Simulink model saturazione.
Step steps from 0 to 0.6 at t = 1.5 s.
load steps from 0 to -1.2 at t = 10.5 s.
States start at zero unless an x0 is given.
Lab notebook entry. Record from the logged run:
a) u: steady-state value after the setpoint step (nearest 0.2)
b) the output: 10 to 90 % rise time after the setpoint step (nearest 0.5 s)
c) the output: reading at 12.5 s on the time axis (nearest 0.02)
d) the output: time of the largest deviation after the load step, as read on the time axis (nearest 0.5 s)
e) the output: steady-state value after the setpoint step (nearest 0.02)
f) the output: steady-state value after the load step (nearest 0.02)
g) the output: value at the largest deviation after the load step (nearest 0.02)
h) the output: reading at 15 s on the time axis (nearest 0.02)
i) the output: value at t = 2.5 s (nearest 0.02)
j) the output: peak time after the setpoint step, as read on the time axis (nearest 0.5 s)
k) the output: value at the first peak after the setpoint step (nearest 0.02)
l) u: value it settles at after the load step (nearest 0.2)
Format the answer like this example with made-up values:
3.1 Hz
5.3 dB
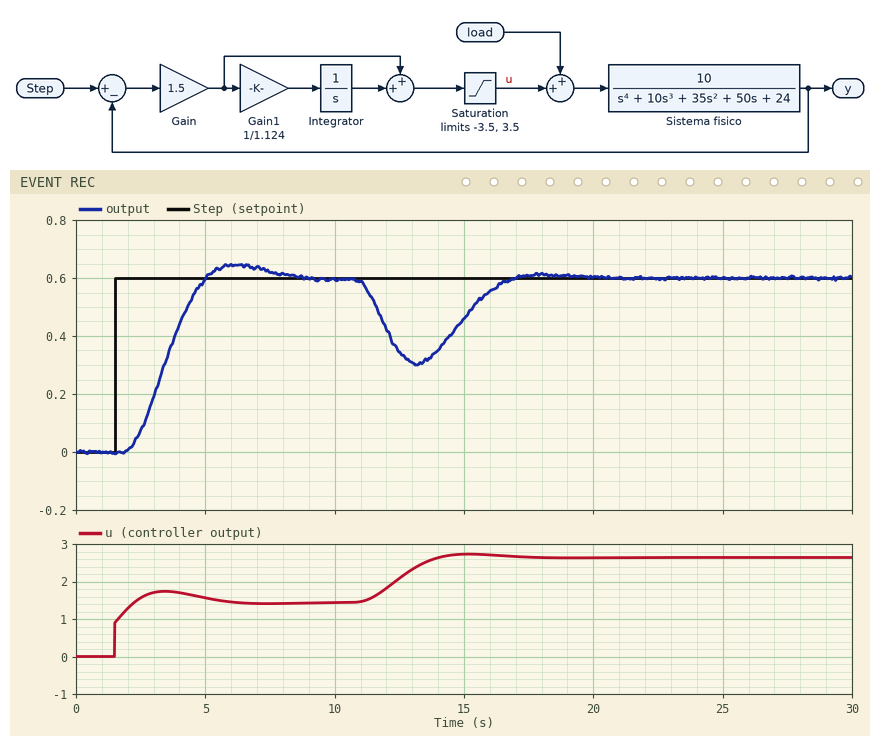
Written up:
1.4
2.0 s
0.34
13.0 s
0.60
0.60
0.30
0.46
0.08
6.0 s
0.64
2.6
